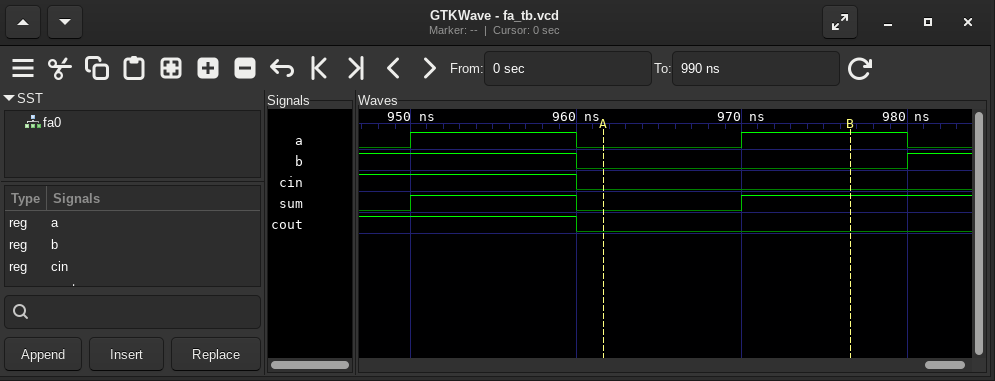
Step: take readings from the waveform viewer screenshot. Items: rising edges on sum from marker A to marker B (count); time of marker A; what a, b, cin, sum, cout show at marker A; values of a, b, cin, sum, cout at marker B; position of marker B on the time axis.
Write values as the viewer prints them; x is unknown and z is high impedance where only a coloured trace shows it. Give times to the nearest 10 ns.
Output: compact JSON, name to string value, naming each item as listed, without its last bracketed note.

{"rising edges on sum from marker A to marker B": "1", "time of marker A": "960 ns", "what a, b, cin, sum, cout show at marker A": "a=0, b=0, cin=0, sum=0, cout=0", "values of a, b, cin, sum, cout at marker B": "a=1, b=0, cin=0, sum=1, cout=0", "position of marker B on the time axis": "980 ns"}
